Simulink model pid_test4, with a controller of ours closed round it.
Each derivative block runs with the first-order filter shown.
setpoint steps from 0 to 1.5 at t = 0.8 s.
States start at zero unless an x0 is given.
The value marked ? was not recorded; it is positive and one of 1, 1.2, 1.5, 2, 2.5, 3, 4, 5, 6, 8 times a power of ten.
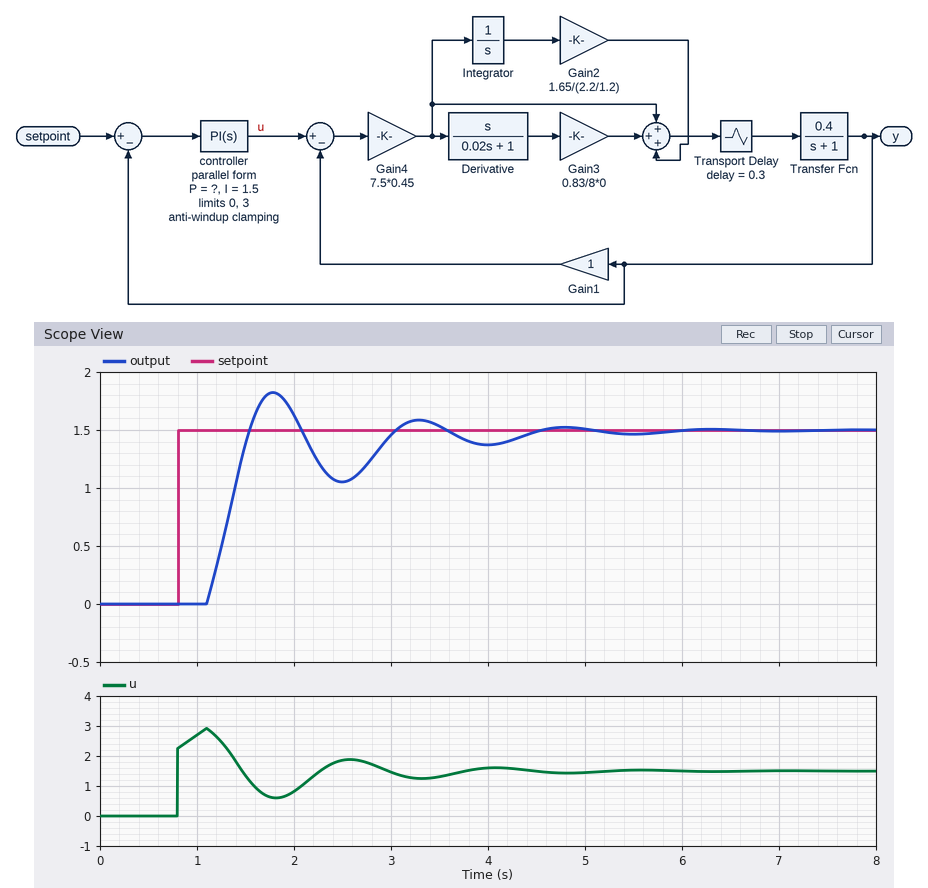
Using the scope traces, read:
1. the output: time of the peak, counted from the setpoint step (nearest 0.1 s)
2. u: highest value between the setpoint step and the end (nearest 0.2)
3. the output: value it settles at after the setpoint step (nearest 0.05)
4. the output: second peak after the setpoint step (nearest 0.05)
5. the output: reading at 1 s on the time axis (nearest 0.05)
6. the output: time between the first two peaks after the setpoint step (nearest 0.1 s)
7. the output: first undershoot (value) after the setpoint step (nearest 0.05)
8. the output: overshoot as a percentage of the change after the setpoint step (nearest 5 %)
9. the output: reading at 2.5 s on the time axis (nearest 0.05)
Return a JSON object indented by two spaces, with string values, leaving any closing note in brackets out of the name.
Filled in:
{
  "the output: time of the peak, counted from the setpoint step": "1.0 s",
  "u: highest value between the setpoint step and the end": "3.0",
  "the output: value it settles at after the setpoint step": "1.50",
  "the output: second peak after the setpoint step": "1.60",
  "the output: reading at 1 s on the time axis": "0.00",
  "the output: time between the first two peaks after the setpoint step": "1.5 s",
  "the output: first undershoot (value) after the setpoint step": "1.05",
  "the output: overshoot as a percentage of the change after the setpoint step": "20 %",
  "the output: reading at 2.5 s on the time axis": "1.05"
}
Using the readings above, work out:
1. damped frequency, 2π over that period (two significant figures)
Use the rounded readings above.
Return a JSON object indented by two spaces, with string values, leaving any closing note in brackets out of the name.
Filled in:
{
  "damped frequency, 2π over that period": "4.2 rad/s"
}
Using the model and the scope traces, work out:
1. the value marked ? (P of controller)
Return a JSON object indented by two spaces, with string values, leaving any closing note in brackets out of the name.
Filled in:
{
  "the value marked ?": "1.5"
}
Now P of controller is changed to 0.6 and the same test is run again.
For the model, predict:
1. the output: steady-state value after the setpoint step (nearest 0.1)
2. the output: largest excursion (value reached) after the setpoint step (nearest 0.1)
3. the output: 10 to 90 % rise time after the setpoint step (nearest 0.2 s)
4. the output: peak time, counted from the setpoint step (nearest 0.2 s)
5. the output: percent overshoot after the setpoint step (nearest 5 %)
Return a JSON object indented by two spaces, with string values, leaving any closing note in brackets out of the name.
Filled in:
{
  "the output: steady-state value after the setpoint step": "1.5",
  "the output: largest excursion (value reached) after the setpoint step": "1.6",
  "the output: 10 to 90 % rise time after the setpoint step": "0.6 s",
  "the output: peak time, counted from the setpoint step": "1.6 s",
  "the output: percent overshoot after the setpoint step": "10 %"
}
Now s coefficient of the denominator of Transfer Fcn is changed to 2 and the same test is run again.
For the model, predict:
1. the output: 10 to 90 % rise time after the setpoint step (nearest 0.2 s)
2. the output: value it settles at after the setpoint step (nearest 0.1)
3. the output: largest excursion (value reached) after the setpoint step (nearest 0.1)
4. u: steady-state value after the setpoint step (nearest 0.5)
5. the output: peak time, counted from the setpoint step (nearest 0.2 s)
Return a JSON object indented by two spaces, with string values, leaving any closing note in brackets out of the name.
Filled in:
{
  "the output: 10 to 90 % rise time after the setpoint step": "0.6 s",
  "the output: value it settles at after the setpoint step": "1.5",
  "the output: largest excursion (value reached) after the setpoint step": "1.8",
  "u: steady-state value after the setpoint step": "1.5",
  "the output: peak time, counted from the setpoint step": "1.6 s"
}
